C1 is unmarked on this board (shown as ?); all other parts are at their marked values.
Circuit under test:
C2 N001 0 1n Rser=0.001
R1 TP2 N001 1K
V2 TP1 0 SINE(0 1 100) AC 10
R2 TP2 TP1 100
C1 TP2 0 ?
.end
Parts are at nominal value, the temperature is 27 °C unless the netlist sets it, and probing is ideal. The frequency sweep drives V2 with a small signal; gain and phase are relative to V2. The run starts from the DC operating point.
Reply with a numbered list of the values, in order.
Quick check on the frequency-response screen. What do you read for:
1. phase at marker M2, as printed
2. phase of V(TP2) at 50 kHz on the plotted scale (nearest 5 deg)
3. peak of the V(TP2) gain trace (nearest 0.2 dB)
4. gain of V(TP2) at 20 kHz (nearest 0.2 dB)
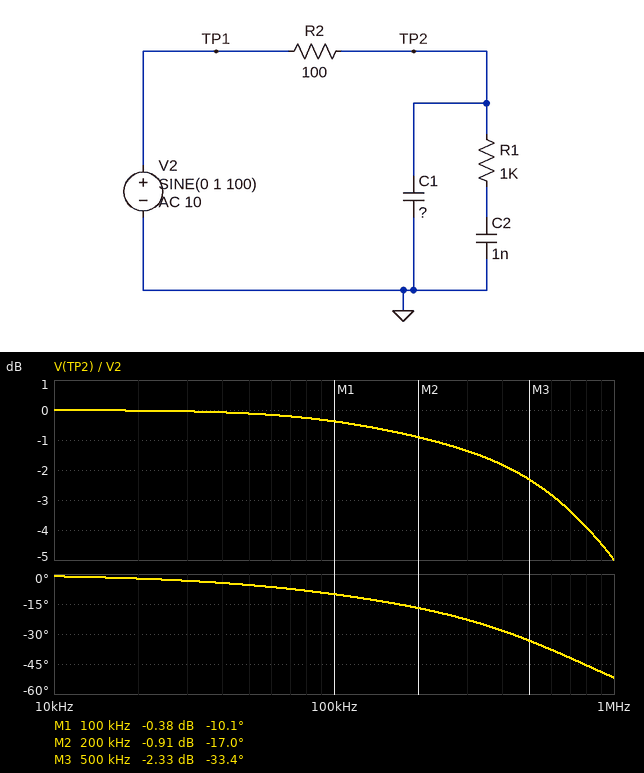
1. -17.0 deg
2. -5 deg
3. 0 dB
4. 0 dB
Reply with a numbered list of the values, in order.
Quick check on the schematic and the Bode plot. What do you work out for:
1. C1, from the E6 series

1. 2.2 nF
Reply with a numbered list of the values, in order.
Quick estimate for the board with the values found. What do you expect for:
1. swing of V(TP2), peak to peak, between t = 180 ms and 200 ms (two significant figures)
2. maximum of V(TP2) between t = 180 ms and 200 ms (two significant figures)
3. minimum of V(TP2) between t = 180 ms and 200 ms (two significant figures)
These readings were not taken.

1. 2.0 V
2. 1.0 V
3. -1.0 V
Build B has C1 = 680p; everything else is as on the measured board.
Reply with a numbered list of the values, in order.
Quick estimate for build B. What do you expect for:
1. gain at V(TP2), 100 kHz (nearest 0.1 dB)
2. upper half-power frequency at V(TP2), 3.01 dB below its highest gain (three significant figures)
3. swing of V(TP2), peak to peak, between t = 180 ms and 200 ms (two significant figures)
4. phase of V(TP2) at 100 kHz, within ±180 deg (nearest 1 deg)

1. -0.3 dB
2. 2.06 MHz
3. 2.0 V
4. -5 deg
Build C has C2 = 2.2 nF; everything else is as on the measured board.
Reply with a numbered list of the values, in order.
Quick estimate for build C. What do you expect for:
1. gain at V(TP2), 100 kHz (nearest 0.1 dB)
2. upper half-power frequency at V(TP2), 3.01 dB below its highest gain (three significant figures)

1. -0.7 dB
2. 636 kHz
